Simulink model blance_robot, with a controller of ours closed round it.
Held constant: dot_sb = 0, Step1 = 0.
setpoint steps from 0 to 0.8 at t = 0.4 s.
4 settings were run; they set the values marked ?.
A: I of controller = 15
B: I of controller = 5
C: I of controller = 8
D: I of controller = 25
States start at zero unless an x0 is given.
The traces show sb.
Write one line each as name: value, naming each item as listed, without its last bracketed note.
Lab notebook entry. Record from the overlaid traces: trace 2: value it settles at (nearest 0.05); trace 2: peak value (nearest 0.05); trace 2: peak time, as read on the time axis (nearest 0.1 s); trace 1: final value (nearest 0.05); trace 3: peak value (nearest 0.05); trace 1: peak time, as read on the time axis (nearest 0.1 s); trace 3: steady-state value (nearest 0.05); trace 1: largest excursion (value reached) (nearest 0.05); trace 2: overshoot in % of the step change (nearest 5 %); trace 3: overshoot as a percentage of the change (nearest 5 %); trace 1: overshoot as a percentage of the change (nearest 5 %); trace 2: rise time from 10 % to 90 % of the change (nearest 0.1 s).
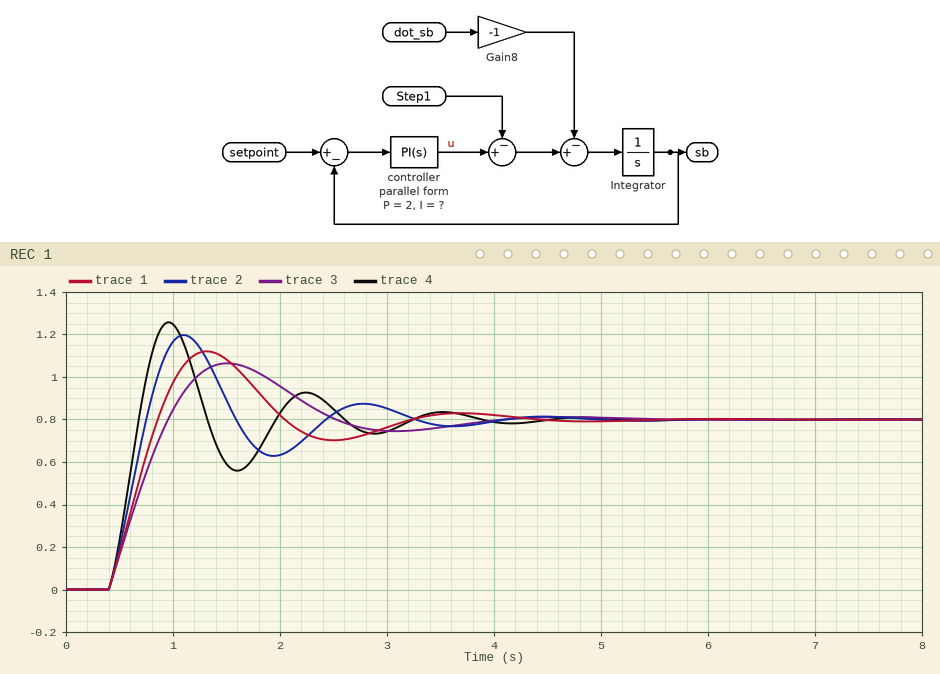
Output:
trace 2: value it settles at: 0.80
trace 2: peak value: 1.20
trace 2: peak time, as read on the time axis: 1.1 s
trace 1: final value: 0.80
trace 3: peak value: 1.05
trace 1: peak time, as read on the time axis: 1.3 s
trace 3: steady-state value: 0.80
trace 1: largest excursion (value reached): 1.10
trace 2: overshoot in % of the step change: 50 %
trace 3: overshoot as a percentage of the change: 35 %
trace 1: overshoot as a percentage of the change: 40 %
trace 2: rise time from 10 % to 90 % of the change: 0.3 s
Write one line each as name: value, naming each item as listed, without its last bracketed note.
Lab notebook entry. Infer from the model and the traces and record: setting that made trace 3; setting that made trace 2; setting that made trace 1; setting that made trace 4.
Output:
setting that made trace 3: B
setting that made trace 2: A
setting that made trace 1: C
setting that made trace 4: D
